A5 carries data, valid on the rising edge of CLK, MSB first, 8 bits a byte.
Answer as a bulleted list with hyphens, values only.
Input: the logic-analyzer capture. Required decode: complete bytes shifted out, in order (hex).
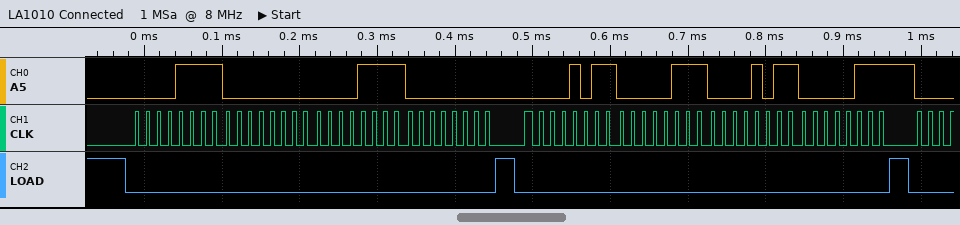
- 0x0F 0x00 0x0F 0x00 0x0B 0x07 0x0B 0x07
